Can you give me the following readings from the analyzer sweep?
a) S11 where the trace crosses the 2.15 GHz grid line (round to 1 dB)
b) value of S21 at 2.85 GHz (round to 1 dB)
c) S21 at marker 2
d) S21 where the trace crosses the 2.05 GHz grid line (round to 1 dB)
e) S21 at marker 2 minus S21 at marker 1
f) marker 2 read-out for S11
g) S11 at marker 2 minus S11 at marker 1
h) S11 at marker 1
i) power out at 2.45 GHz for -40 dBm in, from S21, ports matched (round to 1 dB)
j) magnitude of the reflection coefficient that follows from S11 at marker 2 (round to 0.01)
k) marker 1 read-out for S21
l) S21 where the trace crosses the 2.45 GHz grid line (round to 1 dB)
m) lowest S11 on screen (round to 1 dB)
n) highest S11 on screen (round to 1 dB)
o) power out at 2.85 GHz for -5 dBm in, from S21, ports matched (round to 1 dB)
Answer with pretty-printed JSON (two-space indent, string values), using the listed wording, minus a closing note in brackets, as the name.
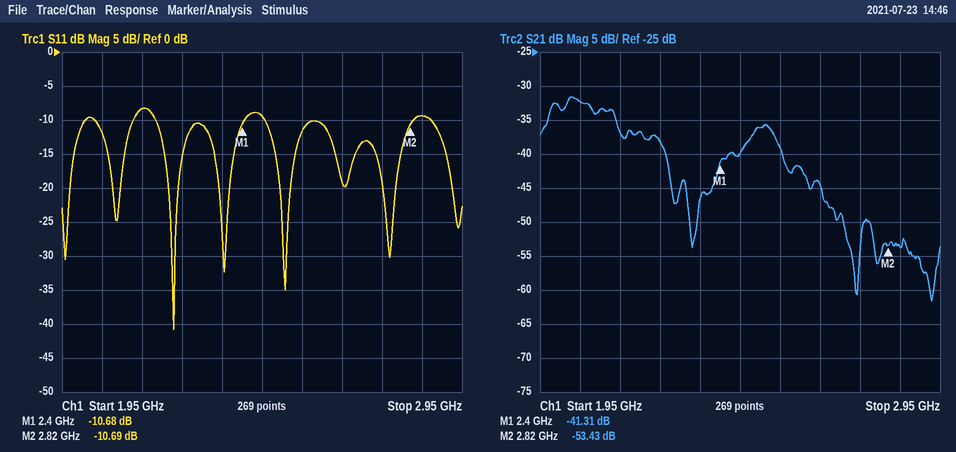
{
  "S11 where the trace crosses the 2.15 GHz grid line": "-8 dB",
  "value of S21 at 2.85 GHz": "-54 dB",
  "S21 at marker 2": "-53.43 dB",
  "S21 where the trace crosses the 2.05 GHz grid line": "-32 dB",
  "S21 at marker 2 minus S21 at marker 1": "-12.12 dB",
  "marker 2 read-out for S11": "-10.69 dB",
  "S11 at marker 2 minus S11 at marker 1": "-0.01 dB",
  "S11 at marker 1": "-10.68 dB",
  "power out at 2.45 GHz for -40 dBm in, from S21, ports matched": "-80 dBm",
  "magnitude of the reflection coefficient that follows from S11 at marker 2": "0.29",
  "marker 1 read-out for S21": "-41.31 dB",
  "S21 where the trace crosses the 2.45 GHz grid line": "-40 dB",
  "lowest S11 on screen": "-41 dB",
  "highest S11 on screen": "-8 dB",
  "power out at 2.85 GHz for -5 dBm in, from S21, ports matched": "-59 dBm"
}
